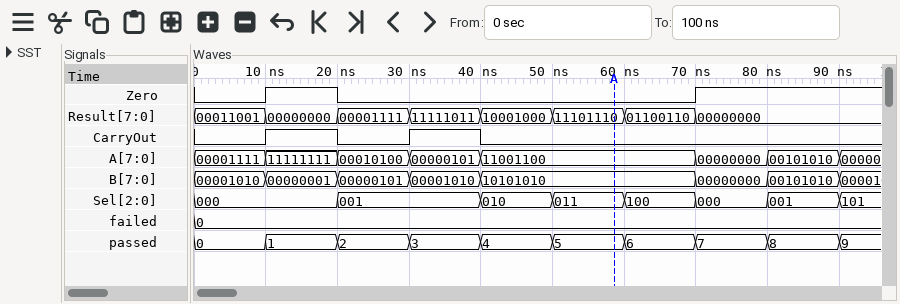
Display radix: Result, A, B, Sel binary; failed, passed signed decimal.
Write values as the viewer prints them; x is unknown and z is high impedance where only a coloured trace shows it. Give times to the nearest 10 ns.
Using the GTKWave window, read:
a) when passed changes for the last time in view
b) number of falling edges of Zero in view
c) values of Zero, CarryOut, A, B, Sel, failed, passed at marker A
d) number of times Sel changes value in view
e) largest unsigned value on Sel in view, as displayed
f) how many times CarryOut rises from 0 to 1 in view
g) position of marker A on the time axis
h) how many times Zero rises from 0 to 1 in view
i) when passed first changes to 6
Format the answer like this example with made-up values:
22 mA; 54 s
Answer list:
90 ns; 1; Zero=0, CarryOut=0, A=11001100, B=10101010, Sel=011, failed=0, passed=5; 7; 101; 2; 60 ns; 2; 60 ns
